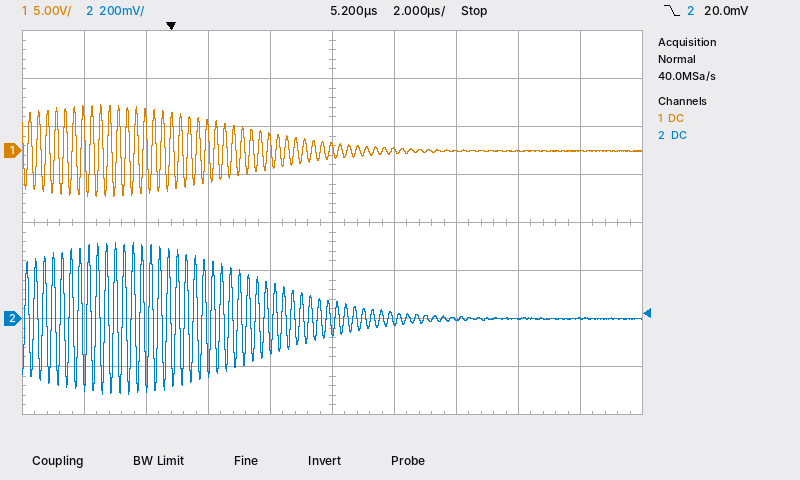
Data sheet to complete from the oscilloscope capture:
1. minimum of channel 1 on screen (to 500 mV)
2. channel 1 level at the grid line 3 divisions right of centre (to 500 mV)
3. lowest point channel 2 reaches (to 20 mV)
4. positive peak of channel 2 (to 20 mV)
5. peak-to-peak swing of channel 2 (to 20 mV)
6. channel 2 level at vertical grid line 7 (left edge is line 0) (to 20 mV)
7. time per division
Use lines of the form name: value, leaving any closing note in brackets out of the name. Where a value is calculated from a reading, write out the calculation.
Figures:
minimum of channel 1 on screen: -5.0 V
channel 1 level at the grid line 3 divisions right of centre: 0.0 V
lowest point channel 2 reaches: -320 mV
positive peak of channel 2: 320 mV
peak-to-peak swing of channel 2: 320 mV − (-320 mV) = 640 mV
channel 2 level at vertical grid line 7 (left edge is line 0): 0 mV
time per division: 2 µs
